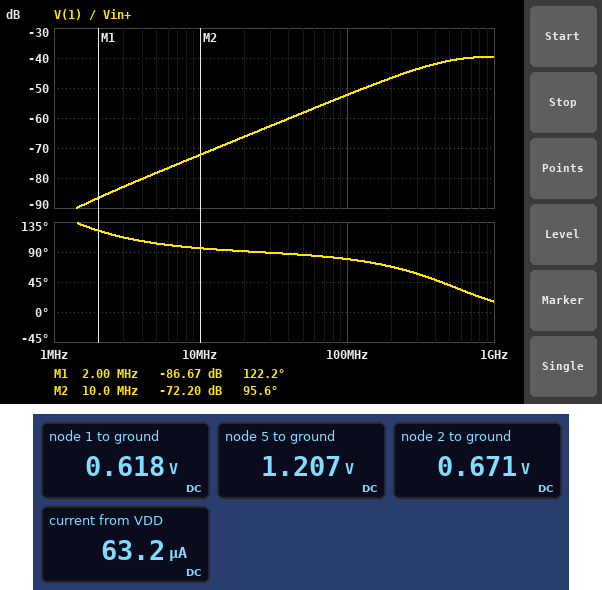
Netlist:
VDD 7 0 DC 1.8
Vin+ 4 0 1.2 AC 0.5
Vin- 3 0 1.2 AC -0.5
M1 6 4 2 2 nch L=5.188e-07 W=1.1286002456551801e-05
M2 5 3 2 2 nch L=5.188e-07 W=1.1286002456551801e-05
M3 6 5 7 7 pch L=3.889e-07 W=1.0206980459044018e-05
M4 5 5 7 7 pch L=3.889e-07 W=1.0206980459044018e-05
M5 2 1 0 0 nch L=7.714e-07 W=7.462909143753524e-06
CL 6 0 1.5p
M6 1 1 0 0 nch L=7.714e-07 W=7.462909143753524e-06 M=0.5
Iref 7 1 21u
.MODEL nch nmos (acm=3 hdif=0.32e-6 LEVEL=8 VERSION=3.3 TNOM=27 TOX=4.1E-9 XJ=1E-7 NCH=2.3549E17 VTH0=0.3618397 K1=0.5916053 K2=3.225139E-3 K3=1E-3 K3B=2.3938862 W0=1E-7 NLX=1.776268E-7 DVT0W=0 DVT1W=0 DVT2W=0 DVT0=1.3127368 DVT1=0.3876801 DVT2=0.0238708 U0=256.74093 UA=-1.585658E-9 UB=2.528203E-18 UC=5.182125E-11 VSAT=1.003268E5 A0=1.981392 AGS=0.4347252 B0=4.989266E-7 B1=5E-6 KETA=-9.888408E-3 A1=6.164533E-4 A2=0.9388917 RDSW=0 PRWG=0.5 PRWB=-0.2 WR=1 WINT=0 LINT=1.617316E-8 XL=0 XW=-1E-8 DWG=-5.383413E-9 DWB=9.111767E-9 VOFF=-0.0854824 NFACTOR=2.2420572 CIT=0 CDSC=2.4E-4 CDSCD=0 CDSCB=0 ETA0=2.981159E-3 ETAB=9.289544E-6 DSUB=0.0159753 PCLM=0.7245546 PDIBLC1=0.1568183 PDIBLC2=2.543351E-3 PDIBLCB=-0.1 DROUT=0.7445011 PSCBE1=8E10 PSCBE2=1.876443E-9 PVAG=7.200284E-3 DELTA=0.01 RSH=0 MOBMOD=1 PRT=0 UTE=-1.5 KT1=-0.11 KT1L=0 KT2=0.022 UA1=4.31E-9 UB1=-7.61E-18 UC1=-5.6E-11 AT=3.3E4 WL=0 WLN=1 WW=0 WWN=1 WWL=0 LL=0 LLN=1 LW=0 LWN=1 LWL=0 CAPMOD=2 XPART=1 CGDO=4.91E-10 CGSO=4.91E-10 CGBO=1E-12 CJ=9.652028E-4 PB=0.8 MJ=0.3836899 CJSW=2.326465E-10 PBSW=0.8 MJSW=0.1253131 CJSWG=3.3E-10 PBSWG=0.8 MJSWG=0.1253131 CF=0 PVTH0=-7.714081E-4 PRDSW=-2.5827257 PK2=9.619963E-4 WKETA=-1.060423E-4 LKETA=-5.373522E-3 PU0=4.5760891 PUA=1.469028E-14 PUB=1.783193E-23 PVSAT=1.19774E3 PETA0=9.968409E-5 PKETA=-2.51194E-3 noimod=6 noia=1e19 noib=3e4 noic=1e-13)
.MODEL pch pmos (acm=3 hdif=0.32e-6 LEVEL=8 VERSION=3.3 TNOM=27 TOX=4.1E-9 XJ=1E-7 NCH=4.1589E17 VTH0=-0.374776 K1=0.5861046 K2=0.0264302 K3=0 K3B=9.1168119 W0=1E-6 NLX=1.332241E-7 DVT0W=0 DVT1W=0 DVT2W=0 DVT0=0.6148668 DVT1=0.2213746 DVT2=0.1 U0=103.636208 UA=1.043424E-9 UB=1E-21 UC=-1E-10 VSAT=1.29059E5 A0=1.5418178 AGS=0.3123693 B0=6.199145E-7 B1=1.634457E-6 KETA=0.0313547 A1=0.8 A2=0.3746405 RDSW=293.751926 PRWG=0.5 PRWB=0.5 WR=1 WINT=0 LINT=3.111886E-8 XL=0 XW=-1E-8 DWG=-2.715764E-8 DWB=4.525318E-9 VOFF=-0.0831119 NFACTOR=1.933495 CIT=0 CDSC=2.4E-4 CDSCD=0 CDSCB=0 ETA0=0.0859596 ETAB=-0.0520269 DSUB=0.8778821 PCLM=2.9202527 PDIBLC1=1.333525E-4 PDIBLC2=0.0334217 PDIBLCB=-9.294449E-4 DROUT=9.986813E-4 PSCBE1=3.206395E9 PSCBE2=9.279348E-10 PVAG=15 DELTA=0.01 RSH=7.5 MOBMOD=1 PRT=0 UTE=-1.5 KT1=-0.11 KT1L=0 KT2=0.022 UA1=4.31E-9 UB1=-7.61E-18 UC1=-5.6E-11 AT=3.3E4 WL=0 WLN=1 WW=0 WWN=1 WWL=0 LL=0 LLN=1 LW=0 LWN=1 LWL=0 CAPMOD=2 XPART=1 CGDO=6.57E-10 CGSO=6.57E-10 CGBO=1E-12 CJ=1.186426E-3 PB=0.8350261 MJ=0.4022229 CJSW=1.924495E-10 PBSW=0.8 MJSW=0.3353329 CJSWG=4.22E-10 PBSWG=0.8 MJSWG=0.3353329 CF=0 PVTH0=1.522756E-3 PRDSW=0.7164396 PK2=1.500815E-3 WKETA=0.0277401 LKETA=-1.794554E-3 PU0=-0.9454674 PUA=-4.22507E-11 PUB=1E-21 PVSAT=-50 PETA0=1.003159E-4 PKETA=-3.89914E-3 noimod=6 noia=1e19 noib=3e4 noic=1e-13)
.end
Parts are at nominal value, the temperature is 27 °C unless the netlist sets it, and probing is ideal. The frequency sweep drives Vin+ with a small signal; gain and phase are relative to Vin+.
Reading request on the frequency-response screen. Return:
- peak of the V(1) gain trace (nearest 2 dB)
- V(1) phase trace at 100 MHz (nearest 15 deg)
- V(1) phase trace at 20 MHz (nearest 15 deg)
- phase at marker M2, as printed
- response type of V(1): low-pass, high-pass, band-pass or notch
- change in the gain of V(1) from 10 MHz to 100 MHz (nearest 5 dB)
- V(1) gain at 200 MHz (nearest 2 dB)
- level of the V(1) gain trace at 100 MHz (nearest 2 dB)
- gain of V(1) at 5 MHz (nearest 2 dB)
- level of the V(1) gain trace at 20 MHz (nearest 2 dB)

-40 dB
75 deg
90 deg
95.6 deg
high-pass
20 dB
-46 dB
-52 dB
-78 dB
-66 dB
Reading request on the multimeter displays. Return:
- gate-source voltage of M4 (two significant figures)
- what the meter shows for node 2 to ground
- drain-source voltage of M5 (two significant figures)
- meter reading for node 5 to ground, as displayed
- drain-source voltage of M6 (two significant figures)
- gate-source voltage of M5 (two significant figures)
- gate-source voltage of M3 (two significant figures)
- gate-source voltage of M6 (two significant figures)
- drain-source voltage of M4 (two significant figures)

-590 mV
0.671 V
670 mV
1.207 V
620 mV
620 mV
-590 mV
620 mV
-590 mV
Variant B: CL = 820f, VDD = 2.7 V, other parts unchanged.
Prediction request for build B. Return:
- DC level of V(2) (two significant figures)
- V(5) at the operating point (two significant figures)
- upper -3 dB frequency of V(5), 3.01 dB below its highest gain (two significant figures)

680 mV
2.1 V
490 MHz
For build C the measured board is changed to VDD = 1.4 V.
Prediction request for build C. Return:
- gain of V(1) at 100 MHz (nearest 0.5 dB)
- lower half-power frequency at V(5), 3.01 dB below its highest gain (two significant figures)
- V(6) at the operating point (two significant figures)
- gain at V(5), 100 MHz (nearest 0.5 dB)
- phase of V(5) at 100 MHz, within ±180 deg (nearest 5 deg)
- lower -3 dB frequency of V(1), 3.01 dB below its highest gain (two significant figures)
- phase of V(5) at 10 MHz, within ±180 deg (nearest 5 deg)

-52.0 dB
1.7 MHz
810 mV
-0.5 dB
-10 deg
340 MHz
5 deg
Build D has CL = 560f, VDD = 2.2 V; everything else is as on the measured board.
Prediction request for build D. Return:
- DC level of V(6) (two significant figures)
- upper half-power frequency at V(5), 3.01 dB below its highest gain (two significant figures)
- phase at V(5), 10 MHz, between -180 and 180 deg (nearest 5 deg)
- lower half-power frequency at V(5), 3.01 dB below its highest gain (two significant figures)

1.6 V
490 MHz
5 deg
1.2 MHz
